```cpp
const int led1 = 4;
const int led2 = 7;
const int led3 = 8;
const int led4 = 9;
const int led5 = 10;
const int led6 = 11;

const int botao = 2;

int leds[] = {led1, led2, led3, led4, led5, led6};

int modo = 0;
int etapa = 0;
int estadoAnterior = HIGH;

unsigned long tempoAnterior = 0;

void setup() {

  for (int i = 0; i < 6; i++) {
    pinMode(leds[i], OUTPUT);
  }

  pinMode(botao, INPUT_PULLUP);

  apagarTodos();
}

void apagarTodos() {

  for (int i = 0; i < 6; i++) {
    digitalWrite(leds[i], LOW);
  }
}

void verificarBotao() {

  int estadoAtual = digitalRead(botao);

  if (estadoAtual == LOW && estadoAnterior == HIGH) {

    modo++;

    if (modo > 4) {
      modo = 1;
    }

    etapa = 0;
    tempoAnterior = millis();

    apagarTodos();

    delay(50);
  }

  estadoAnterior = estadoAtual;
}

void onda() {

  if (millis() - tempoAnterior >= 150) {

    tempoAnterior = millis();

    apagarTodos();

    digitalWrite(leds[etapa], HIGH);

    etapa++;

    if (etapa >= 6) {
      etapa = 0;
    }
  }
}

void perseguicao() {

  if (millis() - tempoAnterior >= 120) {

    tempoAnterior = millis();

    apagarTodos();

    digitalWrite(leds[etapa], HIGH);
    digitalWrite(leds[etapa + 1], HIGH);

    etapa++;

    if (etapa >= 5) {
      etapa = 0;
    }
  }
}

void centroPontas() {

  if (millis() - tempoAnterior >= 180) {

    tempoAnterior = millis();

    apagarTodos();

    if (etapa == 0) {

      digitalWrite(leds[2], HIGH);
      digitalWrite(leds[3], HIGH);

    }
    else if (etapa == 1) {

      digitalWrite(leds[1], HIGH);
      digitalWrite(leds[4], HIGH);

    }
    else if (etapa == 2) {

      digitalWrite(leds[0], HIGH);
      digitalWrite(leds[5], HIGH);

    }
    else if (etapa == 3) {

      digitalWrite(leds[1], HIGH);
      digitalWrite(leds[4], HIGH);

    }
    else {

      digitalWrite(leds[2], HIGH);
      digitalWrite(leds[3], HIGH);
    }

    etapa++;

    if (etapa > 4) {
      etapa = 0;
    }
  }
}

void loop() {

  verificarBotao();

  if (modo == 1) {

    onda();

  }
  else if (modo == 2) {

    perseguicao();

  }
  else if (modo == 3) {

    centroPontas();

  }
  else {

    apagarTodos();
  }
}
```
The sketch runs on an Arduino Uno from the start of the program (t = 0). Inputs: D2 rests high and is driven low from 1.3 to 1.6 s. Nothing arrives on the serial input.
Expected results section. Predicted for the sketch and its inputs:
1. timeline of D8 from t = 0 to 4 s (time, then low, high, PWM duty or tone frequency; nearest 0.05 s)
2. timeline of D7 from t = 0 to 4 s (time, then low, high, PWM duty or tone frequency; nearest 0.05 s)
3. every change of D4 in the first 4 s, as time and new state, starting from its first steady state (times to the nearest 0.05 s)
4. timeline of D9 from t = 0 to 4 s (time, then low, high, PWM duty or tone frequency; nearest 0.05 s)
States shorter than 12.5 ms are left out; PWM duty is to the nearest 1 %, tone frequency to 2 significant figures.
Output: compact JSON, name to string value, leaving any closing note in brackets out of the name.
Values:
{"timeline of D8 from t = 0 to 4 s": "0 s low; 1.75 s high; 1.9 s low; 2.65 s high; 2.8 s low; 3.55 s high; 3.7 s low", "timeline of D7 from t = 0 to 4 s": "0 s low; 1.6 s high; 1.75 s low; 2.5 s high; 2.65 s low; 3.4 s high; 3.55 s low", "every change of D4 in the first 4 s, as time and new state, starting from its first steady state": "0 s low; 1.45 s high; 1.6 s low; 2.35 s high; 2.5 s low; 3.25 s high; 3.4 s low", "timeline of D9 from t = 0 to 4 s": "0 s low; 1.9 s high; 2.05 s low; 2.8 s high; 2.95 s low; 3.7 s high; 3.85 s low"}
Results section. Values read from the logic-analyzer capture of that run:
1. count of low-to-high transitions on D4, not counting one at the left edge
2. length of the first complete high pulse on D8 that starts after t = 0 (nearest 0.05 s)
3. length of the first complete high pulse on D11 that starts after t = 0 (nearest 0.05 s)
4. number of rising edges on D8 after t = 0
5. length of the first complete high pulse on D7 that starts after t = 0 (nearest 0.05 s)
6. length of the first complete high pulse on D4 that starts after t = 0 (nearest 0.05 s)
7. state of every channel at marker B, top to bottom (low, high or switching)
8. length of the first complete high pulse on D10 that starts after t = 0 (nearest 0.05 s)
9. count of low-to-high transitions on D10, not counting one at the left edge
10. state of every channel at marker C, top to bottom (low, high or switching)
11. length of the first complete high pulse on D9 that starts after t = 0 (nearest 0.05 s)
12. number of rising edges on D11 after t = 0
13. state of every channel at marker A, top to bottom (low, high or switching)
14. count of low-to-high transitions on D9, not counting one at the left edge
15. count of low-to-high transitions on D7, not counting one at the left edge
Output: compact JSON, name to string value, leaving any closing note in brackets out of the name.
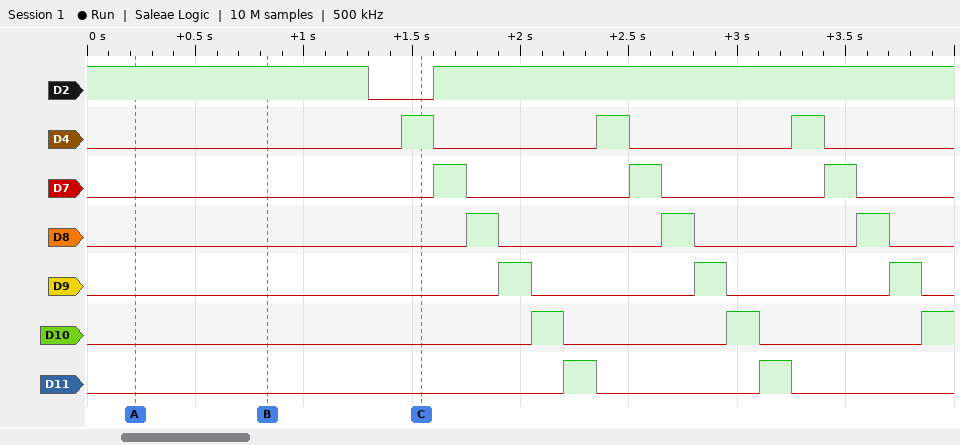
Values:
{"count of low-to-high transitions on D4, not counting one at the left edge": "3", "length of the first complete high pulse on D8 that starts after t = 0": "0.15 s", "length of the first complete high pulse on D11 that starts after t = 0": "0.15 s", "number of rising edges on D8 after t = 0": "3", "length of the first complete high pulse on D7 that starts after t = 0": "0.15 s", "length of the first complete high pulse on D4 that starts after t = 0": "0.15 s", "state of every channel at marker B, top to bottom": "D2 high, D4 low, D7 low, D8 low, D9 low, D10 low, D11 low", "length of the first complete high pulse on D10 that starts after t = 0": "0.15 s", "count of low-to-high transitions on D10, not counting one at the left edge": "3", "state of every channel at marker C, top to bottom": "D2 low, D4 high, D7 low, D8 low, D9 low, D10 low, D11 low", "length of the first complete high pulse on D9 that starts after t = 0": "0.15 s", "number of rising edges on D11 after t = 0": "2", "state of every channel at marker A, top to bottom": "D2 high, D4 low, D7 low, D8 low, D9 low, D10 low, D11 low", "count of low-to-high transitions on D9, not counting one at the left edge": "3", "count of low-to-high transitions on D7, not counting one at the left edge": "3"}
